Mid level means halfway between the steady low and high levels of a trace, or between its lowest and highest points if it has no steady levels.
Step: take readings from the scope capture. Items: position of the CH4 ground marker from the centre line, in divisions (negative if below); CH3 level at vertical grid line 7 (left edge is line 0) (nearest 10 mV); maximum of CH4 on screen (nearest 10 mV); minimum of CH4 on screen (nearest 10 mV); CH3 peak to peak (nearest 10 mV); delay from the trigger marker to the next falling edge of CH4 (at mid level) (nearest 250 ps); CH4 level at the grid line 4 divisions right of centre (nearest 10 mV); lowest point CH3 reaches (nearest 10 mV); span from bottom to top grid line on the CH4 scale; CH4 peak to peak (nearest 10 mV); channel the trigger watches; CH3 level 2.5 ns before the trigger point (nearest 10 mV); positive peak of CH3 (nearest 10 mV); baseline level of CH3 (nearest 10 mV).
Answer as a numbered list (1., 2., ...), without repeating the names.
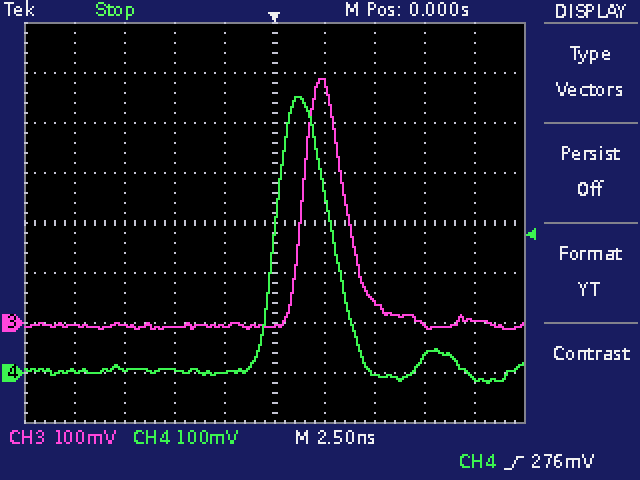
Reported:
1. -3.0 div
2. 40 mV
3. 550 mV
4. -20 mV
5. 500 mV
6. 3.00 ns
7. -10 mV
8. -10 mV
9. 800 mV
10. 570 mV
11. CH4
12. -10 mV
13. 490 mV
14. -10 mV
